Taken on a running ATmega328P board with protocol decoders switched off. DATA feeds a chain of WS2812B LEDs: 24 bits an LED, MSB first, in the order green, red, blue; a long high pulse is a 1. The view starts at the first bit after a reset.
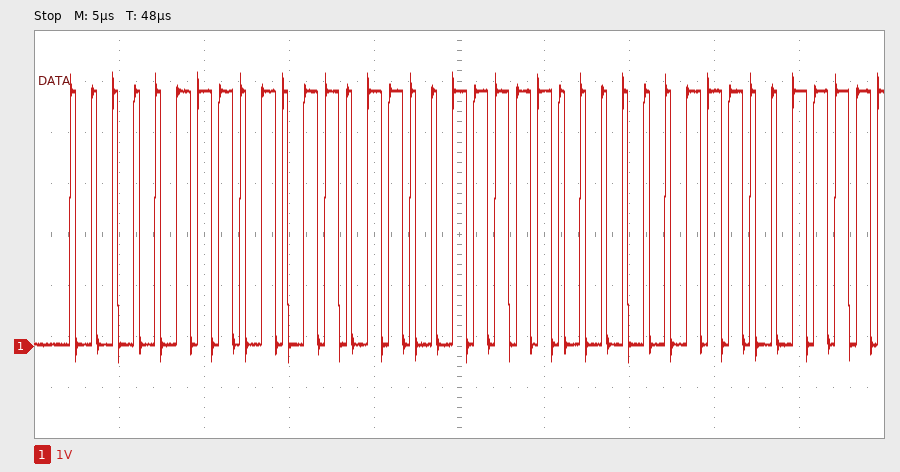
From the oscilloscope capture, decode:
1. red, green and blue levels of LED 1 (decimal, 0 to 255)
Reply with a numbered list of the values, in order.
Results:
1. 91, 7, 62
